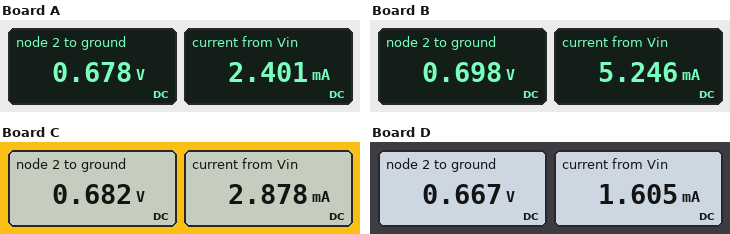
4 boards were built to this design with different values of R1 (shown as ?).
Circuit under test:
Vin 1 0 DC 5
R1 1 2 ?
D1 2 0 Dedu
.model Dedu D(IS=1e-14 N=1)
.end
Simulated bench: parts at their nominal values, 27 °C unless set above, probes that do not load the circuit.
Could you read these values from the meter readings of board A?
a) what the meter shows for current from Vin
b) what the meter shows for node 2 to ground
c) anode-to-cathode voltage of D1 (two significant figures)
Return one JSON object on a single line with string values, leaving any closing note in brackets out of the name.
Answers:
{"what the meter shows for current from Vin": "2.401 mA", "what the meter shows for node 2 to ground": "0.678 V", "anode-to-cathode voltage of D1": "680 mV"}
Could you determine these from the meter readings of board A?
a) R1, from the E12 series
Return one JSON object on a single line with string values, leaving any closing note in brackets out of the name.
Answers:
{"R1, from the E12 series": "1.8 kΩ"}
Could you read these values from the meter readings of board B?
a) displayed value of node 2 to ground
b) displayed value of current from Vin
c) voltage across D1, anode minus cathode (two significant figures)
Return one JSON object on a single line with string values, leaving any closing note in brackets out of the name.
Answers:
{"displayed value of node 2 to ground": "0.698 V", "displayed value of current from Vin": "5.246 mA", "voltage across D1, anode minus cathode": "700 mV"}
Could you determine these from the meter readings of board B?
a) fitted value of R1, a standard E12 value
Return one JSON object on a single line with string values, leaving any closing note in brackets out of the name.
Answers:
{"fitted value of R1, a standard E12 value": "820 Ω"}
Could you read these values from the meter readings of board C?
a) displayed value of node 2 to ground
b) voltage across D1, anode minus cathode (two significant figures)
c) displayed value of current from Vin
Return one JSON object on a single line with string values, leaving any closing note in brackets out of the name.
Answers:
{"displayed value of node 2 to ground": "0.682 V", "voltage across D1, anode minus cathode": "680 mV", "displayed value of current from Vin": "2.878 mA"}
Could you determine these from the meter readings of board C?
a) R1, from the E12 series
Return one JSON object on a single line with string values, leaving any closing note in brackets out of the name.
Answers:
{"R1, from the E12 series": "1.5 kΩ"}
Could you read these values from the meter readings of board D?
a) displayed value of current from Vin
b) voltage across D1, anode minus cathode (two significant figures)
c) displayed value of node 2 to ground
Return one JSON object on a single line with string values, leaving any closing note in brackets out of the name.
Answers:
{"displayed value of current from Vin": "1.605 mA", "voltage across D1, anode minus cathode": "670 mV", "displayed value of node 2 to ground": "0.667 V"}
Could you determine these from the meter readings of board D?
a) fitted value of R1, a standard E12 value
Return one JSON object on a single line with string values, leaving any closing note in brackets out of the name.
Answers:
{"fitted value of R1, a standard E12 value": "2.7 kΩ"}
